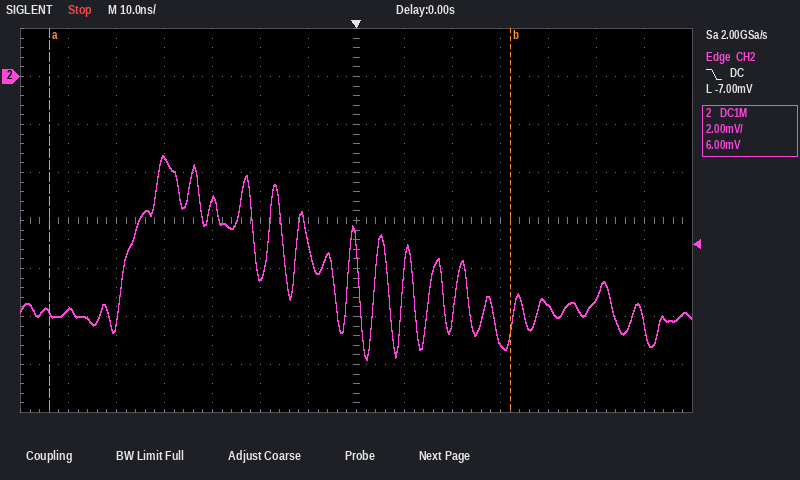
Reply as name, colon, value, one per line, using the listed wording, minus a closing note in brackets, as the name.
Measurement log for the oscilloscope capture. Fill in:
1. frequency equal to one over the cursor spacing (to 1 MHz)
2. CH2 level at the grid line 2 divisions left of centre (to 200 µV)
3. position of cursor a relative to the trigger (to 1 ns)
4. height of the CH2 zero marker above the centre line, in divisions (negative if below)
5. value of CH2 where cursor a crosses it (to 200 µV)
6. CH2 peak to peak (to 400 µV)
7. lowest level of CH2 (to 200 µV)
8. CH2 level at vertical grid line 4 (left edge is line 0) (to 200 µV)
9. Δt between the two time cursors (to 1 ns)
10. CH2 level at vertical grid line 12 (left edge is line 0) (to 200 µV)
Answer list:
frequency equal to one over the cursor spacing: 10 MHz
CH2 level at the grid line 2 divisions left of centre: -8.4 mV
position of cursor a relative to the trigger: -64 ns
height of the CH2 zero marker above the centre line, in divisions: +3.0 div
value of CH2 where cursor a crosses it: -9.8 mV
CH2 peak to peak: 8.4 mV
lowest level of CH2: -11.8 mV
CH2 level at vertical grid line 4 (left edge is line 0): -5.2 mV
Δt between the two time cursors: 96 ns
CH2 level at vertical grid line 12 (left edge is line 0): -9.2 mV
